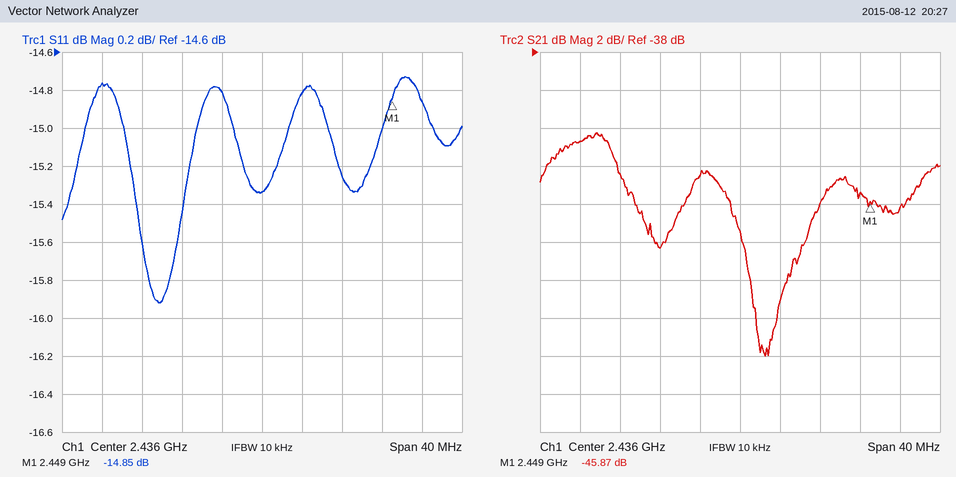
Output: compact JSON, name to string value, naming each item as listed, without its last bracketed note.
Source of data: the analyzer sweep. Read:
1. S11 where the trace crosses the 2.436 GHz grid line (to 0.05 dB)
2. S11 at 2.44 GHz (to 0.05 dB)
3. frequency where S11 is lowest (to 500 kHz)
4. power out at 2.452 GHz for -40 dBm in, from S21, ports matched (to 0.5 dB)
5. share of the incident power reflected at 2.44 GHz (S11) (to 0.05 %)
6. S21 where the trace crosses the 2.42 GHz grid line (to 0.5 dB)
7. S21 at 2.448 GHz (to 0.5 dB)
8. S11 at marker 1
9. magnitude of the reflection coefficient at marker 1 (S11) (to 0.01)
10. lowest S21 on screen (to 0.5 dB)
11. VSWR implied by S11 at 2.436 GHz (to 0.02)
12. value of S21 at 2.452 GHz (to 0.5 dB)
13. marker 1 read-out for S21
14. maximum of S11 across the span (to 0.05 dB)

{"S11 where the trace crosses the 2.436 GHz grid line": "-15.35 dB", "S11 at 2.44 GHz": "-14.80 dB", "frequency where S11 is lowest": "2.4255 GHz", "power out at 2.452 GHz for -40 dBm in, from S21, ports matched": "-86.0 dBm", "share of the incident power reflected at 2.44 GHz (S11)": "3.30 %", "S21 where the trace crosses the 2.42 GHz grid line": "-42.5 dB", "S21 at 2.448 GHz": "-45.5 dB", "S11 at marker 1": "-14.85 dB", "magnitude of the reflection coefficient at marker 1 (S11)": "0.18", "lowest S21 on screen": "-54.0 dB", "VSWR implied by S11 at 2.436 GHz": "1.42", "value of S21 at 2.452 GHz": "-46.0 dB", "marker 1 read-out for S21": "-45.87 dB", "maximum of S11 across the span": "-14.75 dB"}
